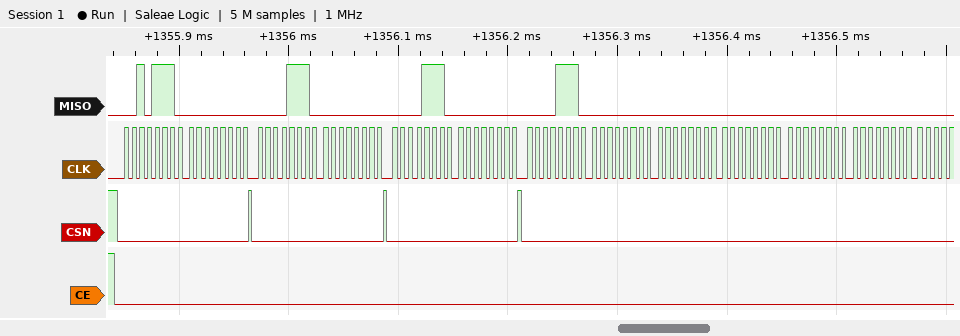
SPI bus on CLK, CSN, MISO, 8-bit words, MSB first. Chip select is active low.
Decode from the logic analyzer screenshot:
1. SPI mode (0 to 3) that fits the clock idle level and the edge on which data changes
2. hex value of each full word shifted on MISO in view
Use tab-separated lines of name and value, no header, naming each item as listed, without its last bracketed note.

SPI mode (0 to 3) that fits the clock idle level and the edge on which data changes	0
hex value of each full word shifted on MISO in view	2E, 00, 0E, 00, 0E, 00, 0E, 00, 00, 00, 00, 00
